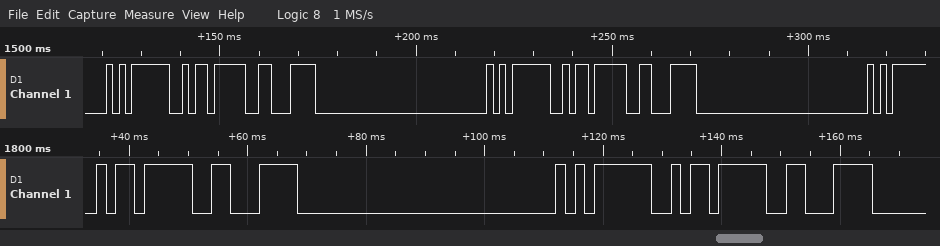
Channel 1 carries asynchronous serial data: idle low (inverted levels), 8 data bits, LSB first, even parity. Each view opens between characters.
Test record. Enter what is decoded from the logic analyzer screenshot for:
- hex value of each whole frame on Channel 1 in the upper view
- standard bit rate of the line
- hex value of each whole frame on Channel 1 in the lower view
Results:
05, 09, 0E, 05, 09, 0E
600 baud
09, 0E, 05, 09, 0E
